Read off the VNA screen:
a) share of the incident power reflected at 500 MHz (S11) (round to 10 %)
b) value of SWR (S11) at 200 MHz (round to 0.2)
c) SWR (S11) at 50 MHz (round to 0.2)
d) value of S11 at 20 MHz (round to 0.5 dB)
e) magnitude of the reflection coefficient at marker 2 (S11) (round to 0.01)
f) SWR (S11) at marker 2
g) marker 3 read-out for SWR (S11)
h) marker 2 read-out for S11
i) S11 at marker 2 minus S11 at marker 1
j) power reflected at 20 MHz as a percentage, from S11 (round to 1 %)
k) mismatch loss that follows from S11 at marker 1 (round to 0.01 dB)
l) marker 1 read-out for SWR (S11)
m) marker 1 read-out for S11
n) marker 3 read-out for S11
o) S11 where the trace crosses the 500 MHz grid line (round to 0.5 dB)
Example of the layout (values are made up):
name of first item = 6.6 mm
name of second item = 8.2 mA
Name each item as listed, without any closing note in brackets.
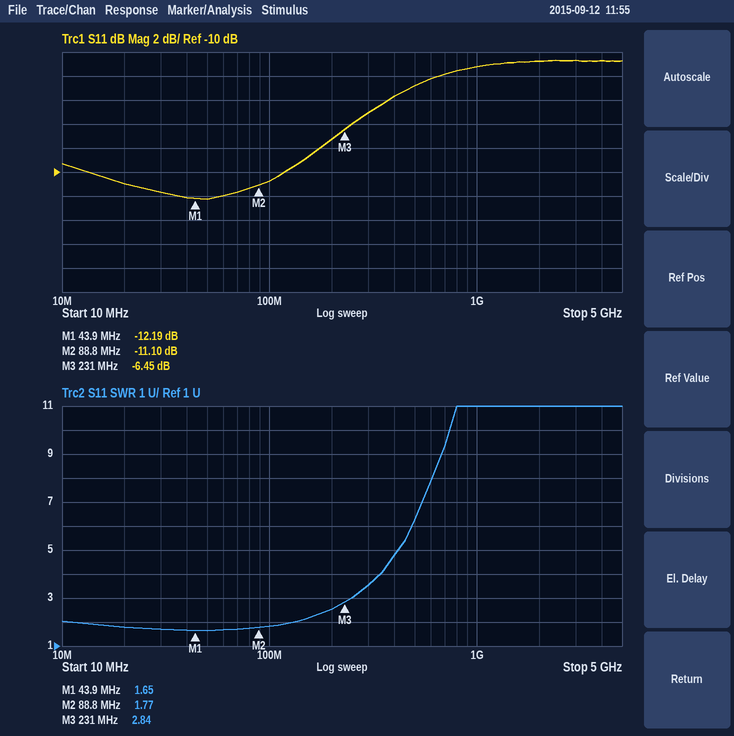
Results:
share of the incident power reflected at 500 MHz (S11) = 50 %
value of SWR (S11) at 200 MHz = 2.6
SWR (S11) at 50 MHz = 1.6
value of S11 at 20 MHz = -11.0 dB
magnitude of the reflection coefficient at marker 2 (S11) = 0.28
SWR (S11) at marker 2 = 1.77
marker 3 read-out for SWR = 2.84
marker 2 read-out for S11 = -11.10 dB
S11 at marker 2 minus S11 at marker 1 = 1.09 dB
power reflected at 20 MHz as a percentage, from S11 = 8 %
mismatch loss that follows from S11 at marker 1 = 0.27 dB
marker 1 read-out for SWR = 1.65
marker 1 read-out for S11 = -12.19 dB
marker 3 read-out for S11 = -6.45 dB
S11 where the trace crosses the 500 MHz grid line = -3.0 dB
